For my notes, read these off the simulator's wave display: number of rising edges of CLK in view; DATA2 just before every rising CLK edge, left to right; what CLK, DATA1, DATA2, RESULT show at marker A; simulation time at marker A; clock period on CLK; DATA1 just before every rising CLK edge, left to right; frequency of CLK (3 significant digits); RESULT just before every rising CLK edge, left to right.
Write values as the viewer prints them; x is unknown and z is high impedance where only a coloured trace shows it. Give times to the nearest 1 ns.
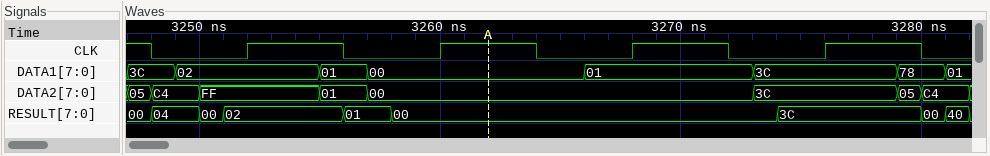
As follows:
4
FF, 00, 00, 3C
CLK=1, DATA1=00, DATA2=00, RESULT=00
3262 ns
8 ns
02, 00, 01, 3C
125 MHz
02, 00, 00, 3C
